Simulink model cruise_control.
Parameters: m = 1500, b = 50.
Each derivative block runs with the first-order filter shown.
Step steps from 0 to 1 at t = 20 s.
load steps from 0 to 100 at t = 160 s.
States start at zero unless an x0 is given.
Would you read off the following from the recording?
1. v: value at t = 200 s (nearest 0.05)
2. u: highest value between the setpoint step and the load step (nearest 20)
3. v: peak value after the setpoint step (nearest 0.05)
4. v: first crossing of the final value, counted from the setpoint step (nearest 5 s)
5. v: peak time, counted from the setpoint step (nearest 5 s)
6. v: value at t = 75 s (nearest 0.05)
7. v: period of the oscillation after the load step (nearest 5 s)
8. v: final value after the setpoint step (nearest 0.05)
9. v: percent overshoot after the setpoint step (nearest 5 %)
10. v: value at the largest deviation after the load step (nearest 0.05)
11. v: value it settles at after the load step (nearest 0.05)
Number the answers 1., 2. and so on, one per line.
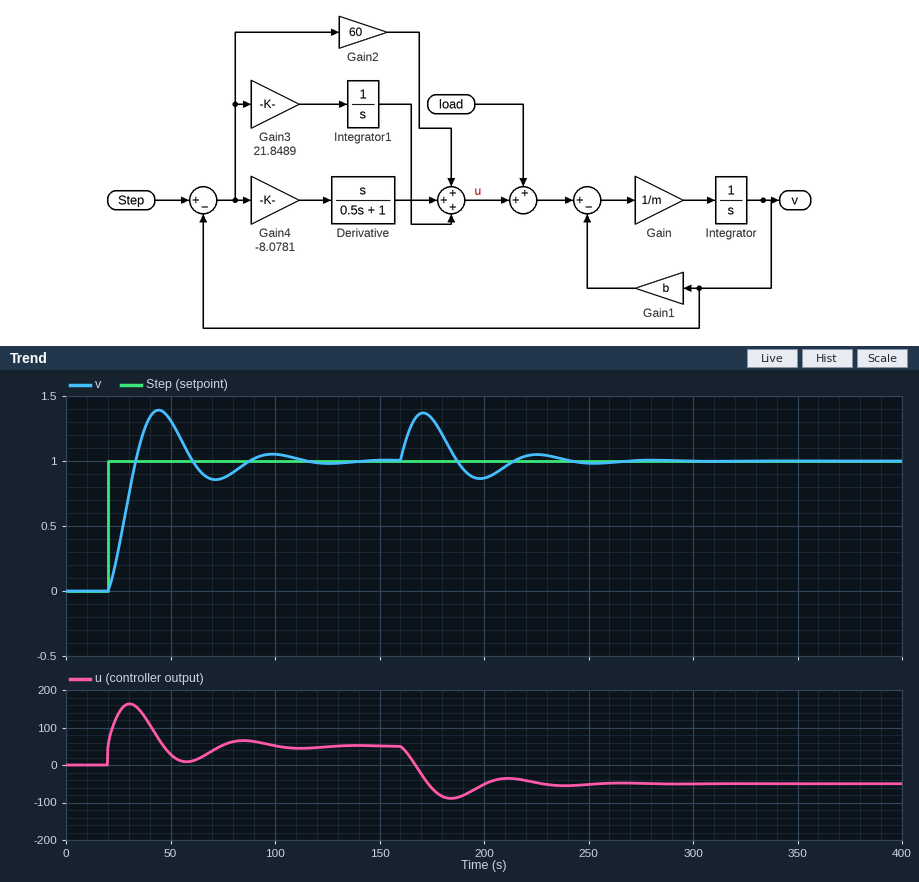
1. 0.85
2. 160
3. 1.40
4. 15 s
5. 25 s
6. 0.85
7. 55 s
8. 1.00
9. 40 %
10. 1.35
11. 1.00
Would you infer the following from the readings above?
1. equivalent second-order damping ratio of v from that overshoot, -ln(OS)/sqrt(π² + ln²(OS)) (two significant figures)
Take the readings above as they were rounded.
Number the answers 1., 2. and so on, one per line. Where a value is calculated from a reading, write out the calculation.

1. ln(0.4) = -0.916; 0.916 / sqrt(9.870 + 0.840) = 0.28
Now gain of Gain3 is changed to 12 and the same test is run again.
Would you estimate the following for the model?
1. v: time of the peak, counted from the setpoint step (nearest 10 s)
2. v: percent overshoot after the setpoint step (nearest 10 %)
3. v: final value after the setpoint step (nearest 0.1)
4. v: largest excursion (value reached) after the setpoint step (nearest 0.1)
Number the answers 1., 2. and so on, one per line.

1. 30 s
2. 30 %
3. 1.0
4. 1.3
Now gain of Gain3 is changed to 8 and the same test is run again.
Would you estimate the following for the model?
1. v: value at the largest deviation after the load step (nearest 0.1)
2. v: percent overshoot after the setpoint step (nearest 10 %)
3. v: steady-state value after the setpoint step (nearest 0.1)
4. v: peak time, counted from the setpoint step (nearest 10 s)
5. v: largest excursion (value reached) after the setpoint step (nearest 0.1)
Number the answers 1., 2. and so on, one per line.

1. 1.5
2. 20 %
3. 1.0
4. 40 s
5. 1.2
